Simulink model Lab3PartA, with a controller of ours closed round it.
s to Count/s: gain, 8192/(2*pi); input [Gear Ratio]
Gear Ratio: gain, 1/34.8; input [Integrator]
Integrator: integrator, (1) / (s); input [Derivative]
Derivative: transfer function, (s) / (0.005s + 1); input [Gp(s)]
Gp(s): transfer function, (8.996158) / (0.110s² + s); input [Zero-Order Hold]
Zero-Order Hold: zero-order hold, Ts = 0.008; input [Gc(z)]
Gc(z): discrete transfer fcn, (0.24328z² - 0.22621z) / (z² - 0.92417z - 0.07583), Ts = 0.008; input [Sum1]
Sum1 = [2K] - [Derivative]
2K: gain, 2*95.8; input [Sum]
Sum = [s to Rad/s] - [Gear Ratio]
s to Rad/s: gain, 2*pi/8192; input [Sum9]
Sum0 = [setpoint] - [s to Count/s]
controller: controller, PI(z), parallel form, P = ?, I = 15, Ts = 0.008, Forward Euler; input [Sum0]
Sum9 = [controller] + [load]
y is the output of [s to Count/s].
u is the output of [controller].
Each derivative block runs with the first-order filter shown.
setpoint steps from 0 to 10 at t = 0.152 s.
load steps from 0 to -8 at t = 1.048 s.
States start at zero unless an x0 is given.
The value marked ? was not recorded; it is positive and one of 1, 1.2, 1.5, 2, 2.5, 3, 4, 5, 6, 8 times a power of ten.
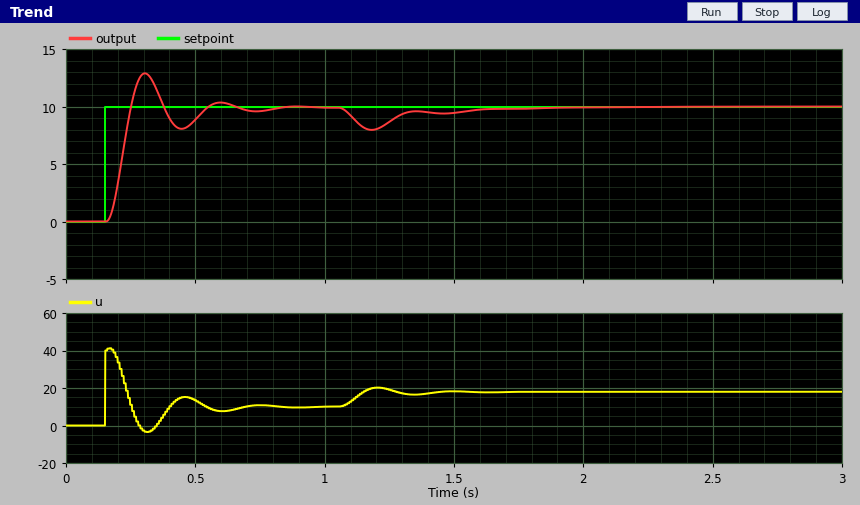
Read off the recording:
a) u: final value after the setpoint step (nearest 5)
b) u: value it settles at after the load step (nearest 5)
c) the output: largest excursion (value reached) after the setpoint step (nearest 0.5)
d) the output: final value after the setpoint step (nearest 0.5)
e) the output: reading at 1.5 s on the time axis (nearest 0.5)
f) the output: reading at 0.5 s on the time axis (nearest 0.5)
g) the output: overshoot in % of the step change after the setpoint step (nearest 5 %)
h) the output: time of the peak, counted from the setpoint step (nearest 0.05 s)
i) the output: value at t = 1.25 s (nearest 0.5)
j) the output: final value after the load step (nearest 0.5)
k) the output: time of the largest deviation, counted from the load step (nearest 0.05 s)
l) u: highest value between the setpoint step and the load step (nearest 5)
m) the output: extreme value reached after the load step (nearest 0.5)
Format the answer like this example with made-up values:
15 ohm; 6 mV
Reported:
10; 20; 13.0; 10.0; 9.5; 9.0; 30 %; 0.15 s; 8.5; 10.0; 0.15 s; 40; 8.0
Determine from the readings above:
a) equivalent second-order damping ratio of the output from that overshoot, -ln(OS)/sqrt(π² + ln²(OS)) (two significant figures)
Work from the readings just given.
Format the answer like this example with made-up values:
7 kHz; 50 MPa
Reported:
0.36
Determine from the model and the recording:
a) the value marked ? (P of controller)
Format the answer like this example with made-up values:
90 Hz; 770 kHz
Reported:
4
